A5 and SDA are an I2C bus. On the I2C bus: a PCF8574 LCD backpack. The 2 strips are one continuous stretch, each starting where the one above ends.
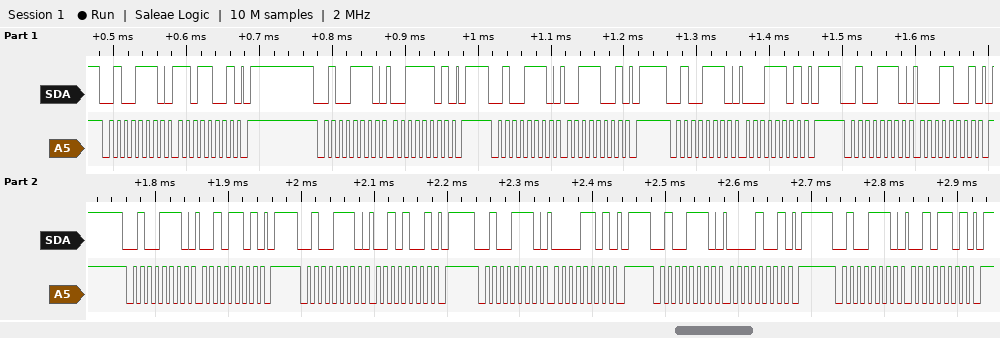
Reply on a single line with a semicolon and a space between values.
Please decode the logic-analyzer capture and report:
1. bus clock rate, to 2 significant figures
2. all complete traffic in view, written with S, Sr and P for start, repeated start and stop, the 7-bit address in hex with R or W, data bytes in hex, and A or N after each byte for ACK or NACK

100 kHz; S 27W A D9 A P S 27W A 3D A P S 27W A 39 A P S 27W A 1D A P S 27W A 19 A P S 27W A 2D A P S 27W A 29 A P S 27W A 0D A P S 27W A 09 A P S 27W A 2D A P
